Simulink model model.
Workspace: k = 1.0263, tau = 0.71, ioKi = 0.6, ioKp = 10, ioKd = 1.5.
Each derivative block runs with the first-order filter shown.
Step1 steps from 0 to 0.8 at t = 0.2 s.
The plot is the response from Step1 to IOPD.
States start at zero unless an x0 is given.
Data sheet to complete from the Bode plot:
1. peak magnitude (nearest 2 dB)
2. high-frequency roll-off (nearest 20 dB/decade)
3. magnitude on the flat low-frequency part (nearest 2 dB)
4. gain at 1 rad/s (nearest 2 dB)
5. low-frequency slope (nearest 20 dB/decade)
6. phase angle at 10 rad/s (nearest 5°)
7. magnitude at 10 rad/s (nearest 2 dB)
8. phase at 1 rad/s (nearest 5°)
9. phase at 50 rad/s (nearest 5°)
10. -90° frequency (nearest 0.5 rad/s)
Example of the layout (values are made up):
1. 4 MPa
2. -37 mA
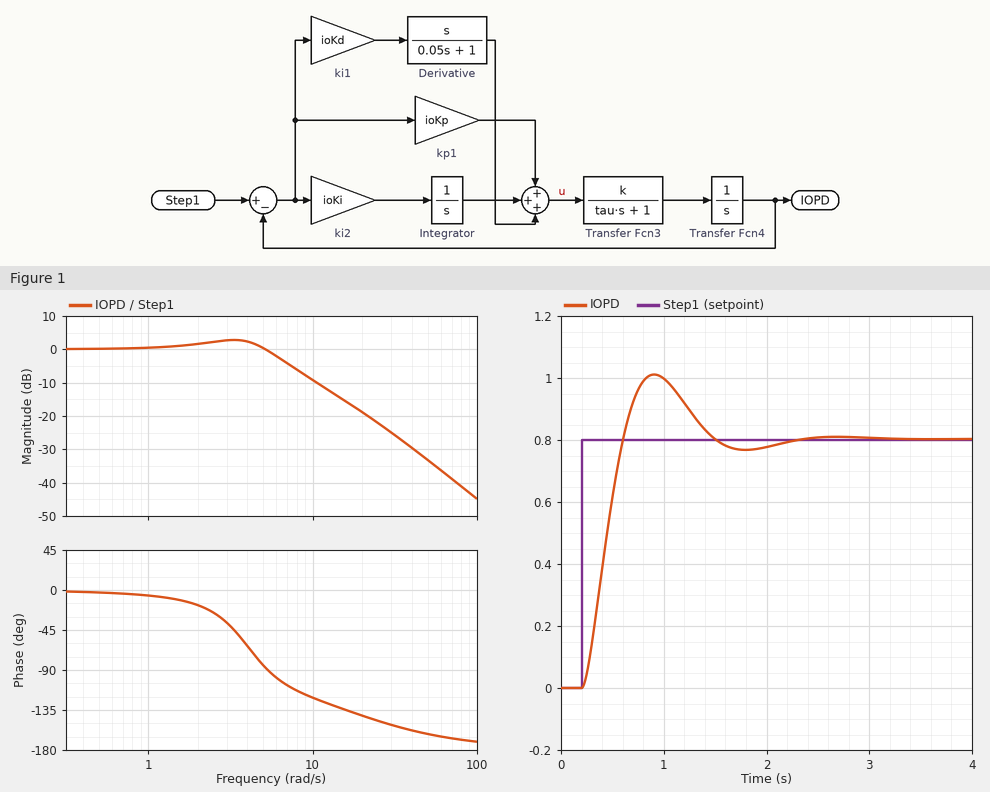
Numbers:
1. 2 dB
2. -40 dB/decade
3. 0 dB
4. 0 dB
5. 0 dB/decade
6. -120°
7. -10 dB
8. -5°
9. -160°
10. 5.5 rad/s
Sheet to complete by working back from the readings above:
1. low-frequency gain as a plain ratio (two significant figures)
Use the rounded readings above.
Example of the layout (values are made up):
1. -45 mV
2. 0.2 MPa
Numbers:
1. 1.0
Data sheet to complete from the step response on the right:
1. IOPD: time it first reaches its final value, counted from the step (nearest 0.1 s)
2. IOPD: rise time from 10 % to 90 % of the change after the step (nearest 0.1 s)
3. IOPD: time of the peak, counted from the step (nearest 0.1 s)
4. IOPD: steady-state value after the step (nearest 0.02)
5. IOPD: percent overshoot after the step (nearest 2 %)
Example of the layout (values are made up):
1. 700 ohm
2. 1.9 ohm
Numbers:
1. 0.4 s
2. 0.3 s
3. 0.7 s
4. 0.80
5. 26 %
